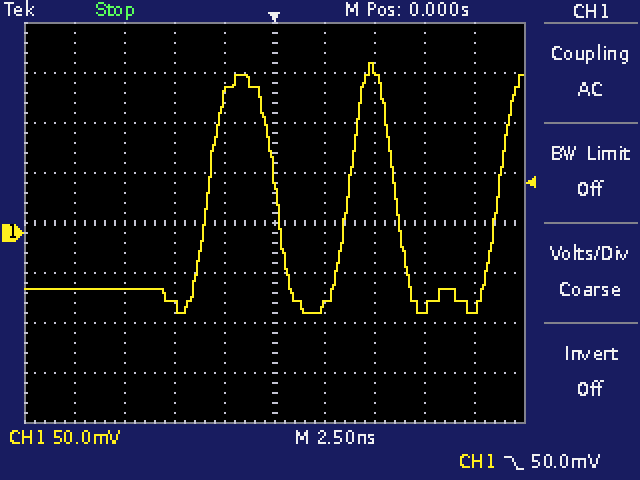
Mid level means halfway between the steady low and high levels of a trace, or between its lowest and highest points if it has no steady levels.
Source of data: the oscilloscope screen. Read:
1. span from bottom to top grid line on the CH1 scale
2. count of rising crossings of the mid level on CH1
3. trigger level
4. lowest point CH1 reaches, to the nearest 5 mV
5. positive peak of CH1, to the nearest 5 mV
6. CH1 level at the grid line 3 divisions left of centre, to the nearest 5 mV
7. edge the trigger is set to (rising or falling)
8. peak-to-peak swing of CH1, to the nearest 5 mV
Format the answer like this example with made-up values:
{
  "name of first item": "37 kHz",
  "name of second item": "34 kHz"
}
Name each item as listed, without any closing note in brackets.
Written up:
{
  "span from bottom to top grid line on the CH1 scale": "400 mV",
  "count of rising crossings of the mid level on CH1": "3",
  "trigger level": "50.0 mV",
  "lowest point CH1 reaches, to the nearest 5 mV": "-80 mV",
  "positive peak of CH1, to the nearest 5 mV": "170 mV",
  "CH1 level at the grid line 3 divisions left of centre, to the nearest 5 mV": "-55 mV",
  "edge the trigger is set to": "falling",
  "peak-to-peak swing of CH1, to the nearest 5 mV": "250 mV"
}
